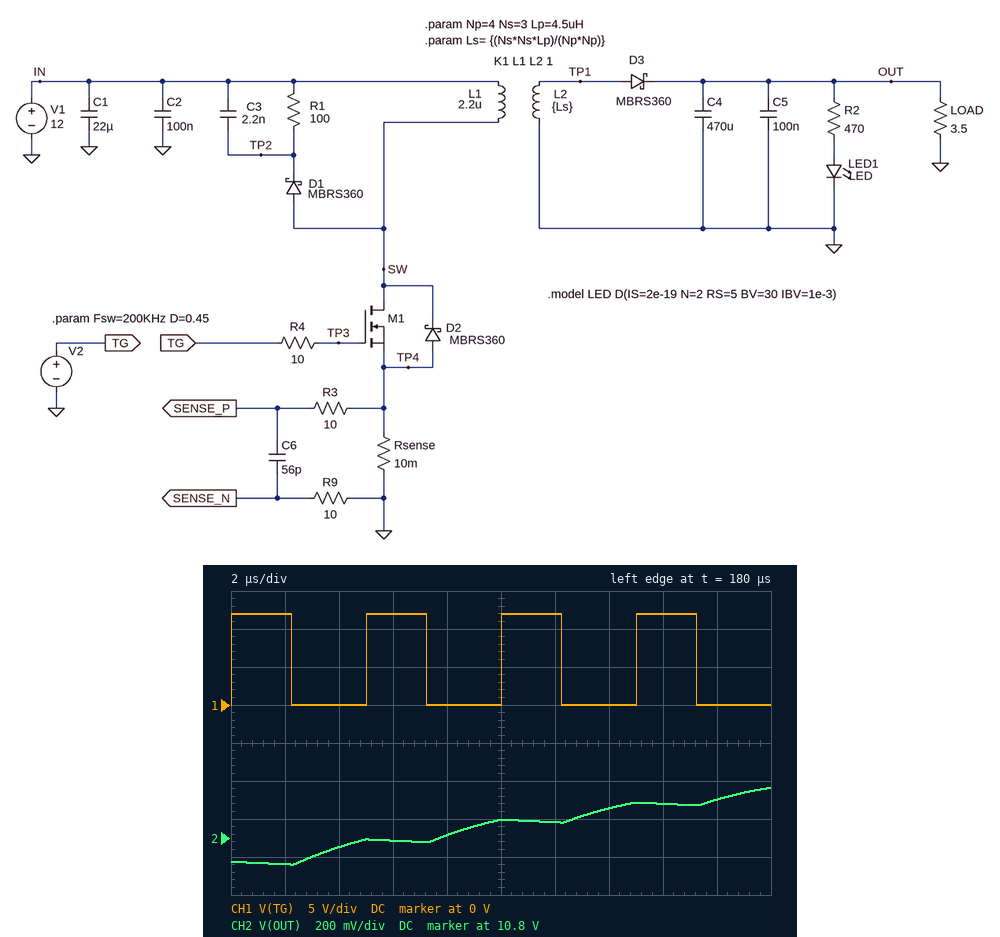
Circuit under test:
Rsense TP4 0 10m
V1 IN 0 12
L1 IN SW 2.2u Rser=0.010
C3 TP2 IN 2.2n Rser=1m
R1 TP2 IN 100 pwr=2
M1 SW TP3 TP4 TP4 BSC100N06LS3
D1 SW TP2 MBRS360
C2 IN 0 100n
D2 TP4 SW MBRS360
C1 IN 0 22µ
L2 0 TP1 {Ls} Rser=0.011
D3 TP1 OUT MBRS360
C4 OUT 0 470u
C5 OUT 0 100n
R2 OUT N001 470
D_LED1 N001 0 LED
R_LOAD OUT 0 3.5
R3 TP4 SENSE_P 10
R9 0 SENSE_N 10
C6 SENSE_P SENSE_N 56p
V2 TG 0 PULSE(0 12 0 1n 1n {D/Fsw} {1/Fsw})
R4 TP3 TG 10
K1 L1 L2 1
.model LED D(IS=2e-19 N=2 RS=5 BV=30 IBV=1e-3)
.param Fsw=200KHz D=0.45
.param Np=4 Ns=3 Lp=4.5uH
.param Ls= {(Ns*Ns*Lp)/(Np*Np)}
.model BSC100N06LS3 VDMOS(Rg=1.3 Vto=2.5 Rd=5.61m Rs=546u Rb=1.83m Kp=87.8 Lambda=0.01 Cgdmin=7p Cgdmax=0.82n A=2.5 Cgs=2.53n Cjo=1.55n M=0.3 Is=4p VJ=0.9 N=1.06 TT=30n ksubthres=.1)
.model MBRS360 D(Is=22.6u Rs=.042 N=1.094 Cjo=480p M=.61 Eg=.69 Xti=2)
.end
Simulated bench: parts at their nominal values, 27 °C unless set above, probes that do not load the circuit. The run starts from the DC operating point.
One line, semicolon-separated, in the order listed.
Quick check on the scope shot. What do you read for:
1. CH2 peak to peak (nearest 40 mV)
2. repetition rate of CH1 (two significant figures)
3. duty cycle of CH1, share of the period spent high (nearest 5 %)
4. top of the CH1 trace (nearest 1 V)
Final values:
400 mV; 200 kHz; 45 %; 12 V
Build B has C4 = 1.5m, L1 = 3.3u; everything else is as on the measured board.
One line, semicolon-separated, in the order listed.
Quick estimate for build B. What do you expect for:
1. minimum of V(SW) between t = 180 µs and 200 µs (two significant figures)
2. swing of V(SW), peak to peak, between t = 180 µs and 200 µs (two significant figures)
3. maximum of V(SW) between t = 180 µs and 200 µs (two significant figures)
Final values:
1.0 V; 21 V; 22 V
